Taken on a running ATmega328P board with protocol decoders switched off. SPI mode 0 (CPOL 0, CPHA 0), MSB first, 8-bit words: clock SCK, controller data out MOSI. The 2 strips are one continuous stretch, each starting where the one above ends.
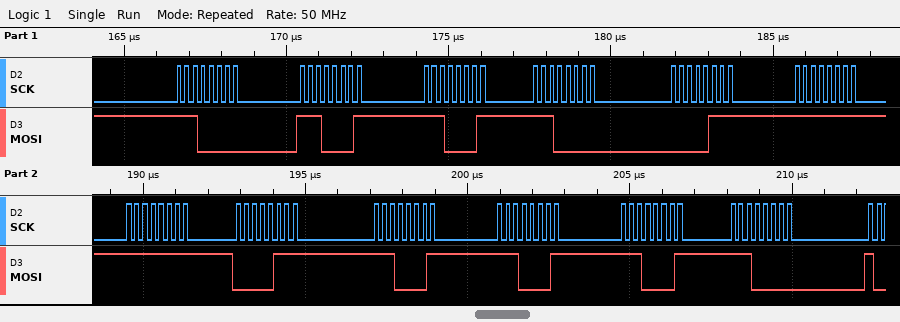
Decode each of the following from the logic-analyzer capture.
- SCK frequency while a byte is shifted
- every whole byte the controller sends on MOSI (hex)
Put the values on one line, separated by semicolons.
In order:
4 MHz; E0 E1 E1 E0 07 FF FF 07 E1 E1 E1 E0
